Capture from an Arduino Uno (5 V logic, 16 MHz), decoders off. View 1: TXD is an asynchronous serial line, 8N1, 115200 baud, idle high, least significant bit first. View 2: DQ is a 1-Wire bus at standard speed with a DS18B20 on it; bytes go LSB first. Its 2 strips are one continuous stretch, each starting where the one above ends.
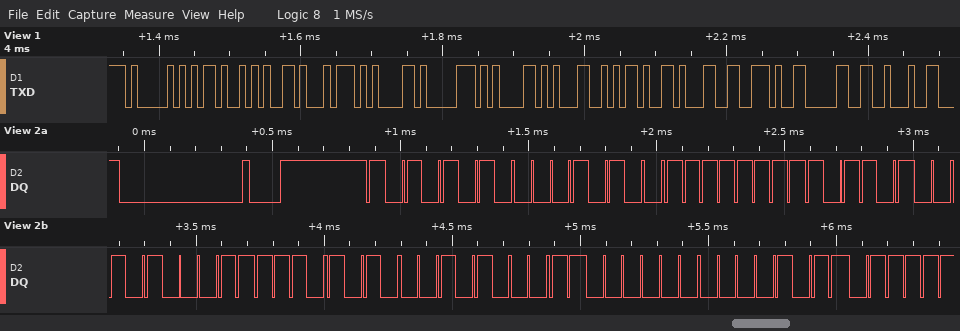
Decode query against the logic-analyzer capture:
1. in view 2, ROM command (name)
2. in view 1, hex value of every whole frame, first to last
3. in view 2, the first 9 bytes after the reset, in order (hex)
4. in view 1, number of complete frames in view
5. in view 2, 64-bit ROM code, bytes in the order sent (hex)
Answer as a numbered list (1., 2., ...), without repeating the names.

1. Match ROM
2. 41 2D 65 74 61 70 61 31 2D 31 2E 30 22
3. 55 28 FF 2D C5 57 14 03 D0
4. 13
5. 28 FF 2D C5 57 14 03 D0
